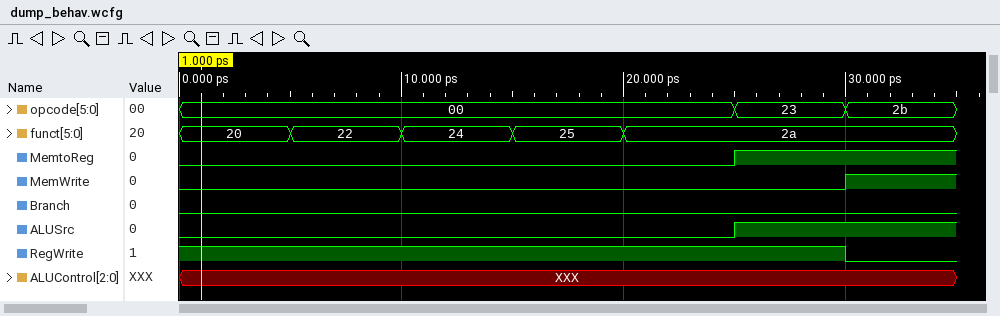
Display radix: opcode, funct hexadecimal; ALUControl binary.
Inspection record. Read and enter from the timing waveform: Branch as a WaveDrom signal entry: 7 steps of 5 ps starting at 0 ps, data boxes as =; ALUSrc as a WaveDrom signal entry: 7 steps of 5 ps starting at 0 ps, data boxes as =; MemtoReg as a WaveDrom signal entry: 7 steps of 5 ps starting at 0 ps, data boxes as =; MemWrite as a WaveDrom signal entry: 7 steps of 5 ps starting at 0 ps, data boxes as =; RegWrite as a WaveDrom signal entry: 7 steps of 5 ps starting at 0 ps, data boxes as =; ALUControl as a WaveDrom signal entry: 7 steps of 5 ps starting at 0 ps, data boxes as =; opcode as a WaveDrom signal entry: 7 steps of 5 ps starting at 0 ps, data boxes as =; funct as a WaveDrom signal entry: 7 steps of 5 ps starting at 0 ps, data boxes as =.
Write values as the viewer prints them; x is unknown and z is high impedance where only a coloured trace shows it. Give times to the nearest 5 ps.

{name: 'Branch', wave: '0......'}
{name: 'ALUSrc', wave: '0....1.'}
{name: 'MemtoReg', wave: '0....1.'}
{name: 'MemWrite', wave: '0.....1'}
{name: 'RegWrite', wave: '1.....0'}
{name: 'ALUControl', wave: 'x......'}
{name: 'opcode', wave: '=....==', data: '00 23 2b'}
{name: 'funct', wave: '=====..', data: '20 22 24 25 2a'}
